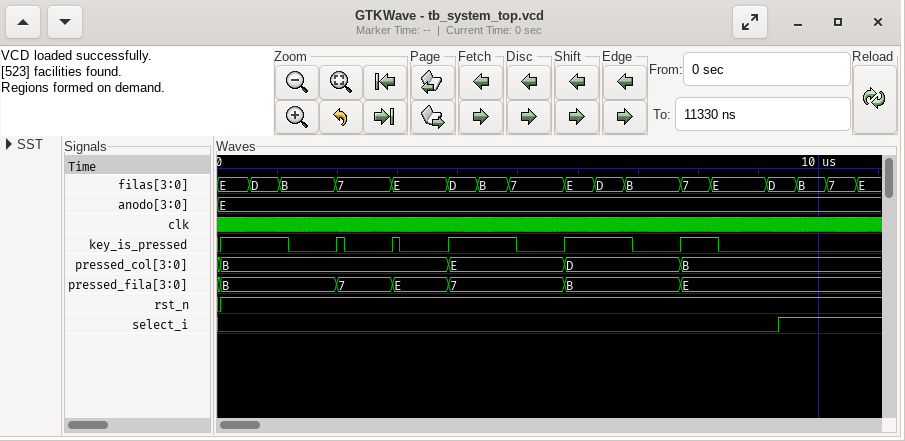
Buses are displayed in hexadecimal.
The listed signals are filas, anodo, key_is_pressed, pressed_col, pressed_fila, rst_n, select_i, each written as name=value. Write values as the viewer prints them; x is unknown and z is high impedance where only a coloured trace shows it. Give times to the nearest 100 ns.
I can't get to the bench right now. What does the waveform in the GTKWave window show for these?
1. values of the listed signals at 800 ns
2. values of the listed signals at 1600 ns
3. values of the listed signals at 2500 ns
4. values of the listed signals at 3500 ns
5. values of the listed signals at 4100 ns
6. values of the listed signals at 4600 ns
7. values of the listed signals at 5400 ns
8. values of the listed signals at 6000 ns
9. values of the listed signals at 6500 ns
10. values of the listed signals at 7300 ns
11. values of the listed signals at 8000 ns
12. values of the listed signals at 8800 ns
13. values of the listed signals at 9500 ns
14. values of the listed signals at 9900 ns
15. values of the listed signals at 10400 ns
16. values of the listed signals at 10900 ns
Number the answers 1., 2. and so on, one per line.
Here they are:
1. filas=D, anodo=E, key_is_pressed=1, pressed_col=B, pressed_fila=B, rst_n=1, select_i=0
2. filas=B, anodo=E, key_is_pressed=0, pressed_col=B, pressed_fila=B, rst_n=1, select_i=0
3. filas=7, anodo=E, key_is_pressed=0, pressed_col=B, pressed_fila=7, rst_n=1, select_i=0
4. filas=E, anodo=E, key_is_pressed=0, pressed_col=B, pressed_fila=E, rst_n=1, select_i=0
5. filas=D, anodo=E, key_is_pressed=1, pressed_col=E, pressed_fila=7, rst_n=1, select_i=0
6. filas=B, anodo=E, key_is_pressed=1, pressed_col=E, pressed_fila=7, rst_n=1, select_i=0
7. filas=7, anodo=E, key_is_pressed=0, pressed_col=E, pressed_fila=7, rst_n=1, select_i=0
8. filas=E, anodo=E, key_is_pressed=1, pressed_col=D, pressed_fila=B, rst_n=1, select_i=0
9. filas=D, anodo=E, key_is_pressed=1, pressed_col=D, pressed_fila=B, rst_n=1, select_i=0
10. filas=B, anodo=E, key_is_pressed=0, pressed_col=D, pressed_fila=B, rst_n=1, select_i=0
11. filas=7, anodo=E, key_is_pressed=1, pressed_col=B, pressed_fila=E, rst_n=1, select_i=0
12. filas=E, anodo=E, key_is_pressed=0, pressed_col=B, pressed_fila=E, rst_n=1, select_i=0
13. filas=D, anodo=E, key_is_pressed=0, pressed_col=B, pressed_fila=E, rst_n=1, select_i=1
14. filas=B, anodo=E, key_is_pressed=0, pressed_col=B, pressed_fila=E, rst_n=1, select_i=1
15. filas=7, anodo=E, key_is_pressed=0, pressed_col=B, pressed_fila=E, rst_n=1, select_i=1
16. filas=E, anodo=E, key_is_pressed=0, pressed_col=B, pressed_fila=E, rst_n=1, select_i=1
